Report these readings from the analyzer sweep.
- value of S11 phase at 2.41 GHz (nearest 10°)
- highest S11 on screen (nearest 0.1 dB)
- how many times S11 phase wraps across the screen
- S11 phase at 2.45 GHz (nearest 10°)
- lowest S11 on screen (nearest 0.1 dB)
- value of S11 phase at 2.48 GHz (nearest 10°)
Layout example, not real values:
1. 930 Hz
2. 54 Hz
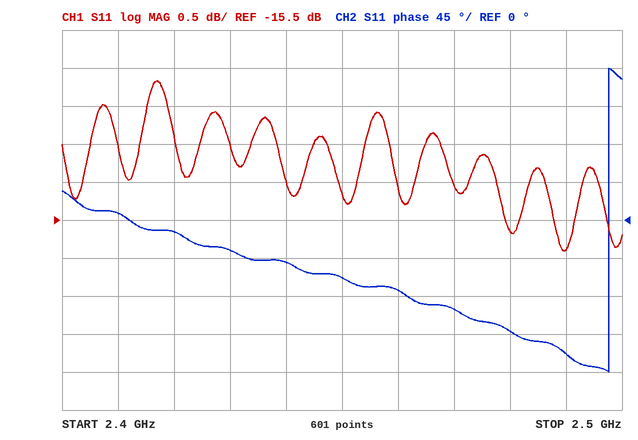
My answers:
1. 10°
2. -13.7 dB
3. 1
4. -70°
5. -15.9 dB
6. -130°
